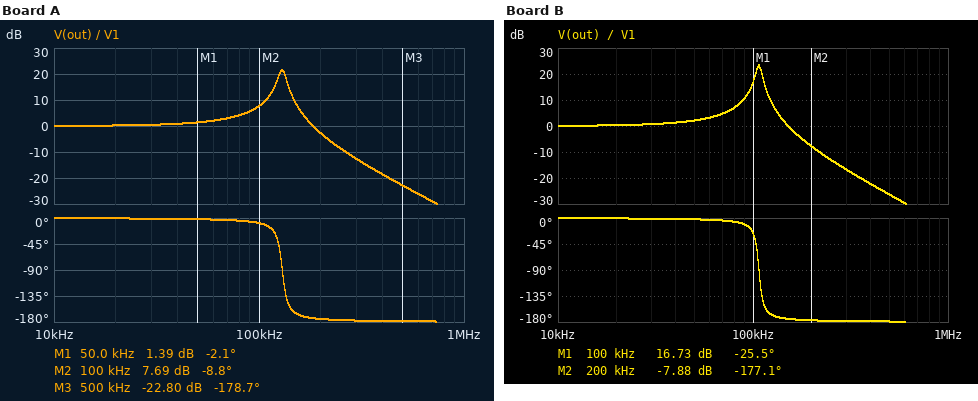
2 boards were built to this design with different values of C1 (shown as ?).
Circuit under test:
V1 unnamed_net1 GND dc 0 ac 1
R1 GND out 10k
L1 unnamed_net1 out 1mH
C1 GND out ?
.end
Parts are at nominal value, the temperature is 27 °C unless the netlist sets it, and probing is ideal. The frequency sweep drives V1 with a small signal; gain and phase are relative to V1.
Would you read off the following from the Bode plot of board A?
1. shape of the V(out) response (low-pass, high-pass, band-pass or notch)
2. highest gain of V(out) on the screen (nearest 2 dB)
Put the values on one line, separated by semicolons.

low-pass; 22 dB
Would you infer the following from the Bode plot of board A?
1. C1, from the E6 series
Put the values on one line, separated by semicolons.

1.5 nF
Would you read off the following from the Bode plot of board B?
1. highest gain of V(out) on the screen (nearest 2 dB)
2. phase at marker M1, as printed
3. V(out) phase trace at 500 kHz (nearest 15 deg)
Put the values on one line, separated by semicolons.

24 dB; -25.5 deg; -180 deg
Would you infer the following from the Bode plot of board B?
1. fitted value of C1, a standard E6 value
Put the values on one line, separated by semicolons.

2.2 nF
